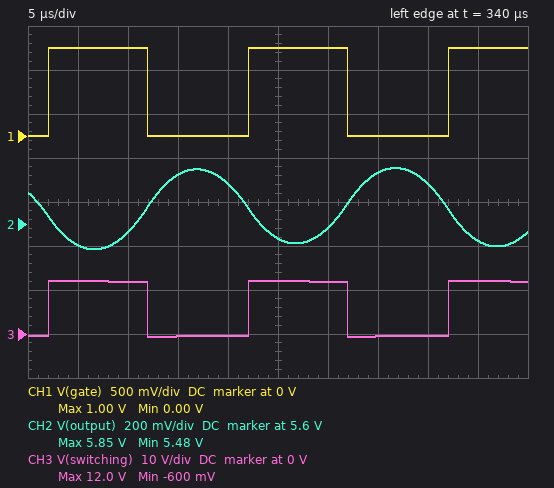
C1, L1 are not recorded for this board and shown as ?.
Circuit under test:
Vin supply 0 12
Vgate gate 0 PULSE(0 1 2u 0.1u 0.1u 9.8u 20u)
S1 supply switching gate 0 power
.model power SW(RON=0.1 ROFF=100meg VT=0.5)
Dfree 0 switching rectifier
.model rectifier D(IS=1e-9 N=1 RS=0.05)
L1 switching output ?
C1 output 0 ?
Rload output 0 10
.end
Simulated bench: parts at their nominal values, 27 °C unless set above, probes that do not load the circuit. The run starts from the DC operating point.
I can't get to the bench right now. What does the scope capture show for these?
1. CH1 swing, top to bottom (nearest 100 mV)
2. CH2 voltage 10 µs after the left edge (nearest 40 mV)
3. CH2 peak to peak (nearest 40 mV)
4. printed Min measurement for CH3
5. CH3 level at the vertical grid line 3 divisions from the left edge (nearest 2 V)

1.0 V
5.56 V
360 mV
-600 mV
0 V
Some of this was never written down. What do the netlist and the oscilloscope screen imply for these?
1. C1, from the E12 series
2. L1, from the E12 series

6.8 µF
68 µH
